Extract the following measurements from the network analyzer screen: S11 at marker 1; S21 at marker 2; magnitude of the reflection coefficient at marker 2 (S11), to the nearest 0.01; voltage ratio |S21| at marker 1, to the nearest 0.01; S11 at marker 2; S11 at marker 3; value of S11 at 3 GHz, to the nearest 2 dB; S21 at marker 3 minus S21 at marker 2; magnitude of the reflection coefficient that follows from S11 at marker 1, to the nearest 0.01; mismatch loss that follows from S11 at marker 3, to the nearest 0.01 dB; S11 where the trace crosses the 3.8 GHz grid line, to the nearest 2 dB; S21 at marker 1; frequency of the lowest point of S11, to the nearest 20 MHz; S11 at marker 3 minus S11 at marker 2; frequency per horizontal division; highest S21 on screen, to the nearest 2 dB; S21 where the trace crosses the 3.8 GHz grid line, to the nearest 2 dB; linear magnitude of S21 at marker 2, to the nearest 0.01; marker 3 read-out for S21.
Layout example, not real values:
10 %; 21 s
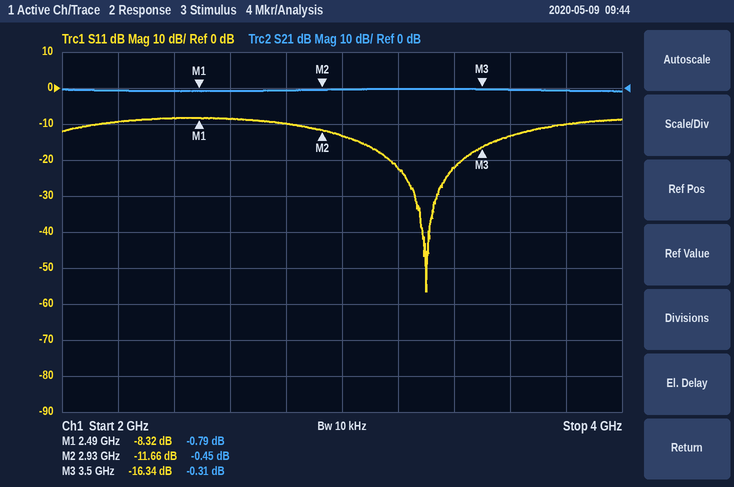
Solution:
-8.32 dB; -0.45 dB; 0.26; 0.91; -11.66 dB; -16.34 dB; -14 dB; 0.14 dB; 0.38; 0.10 dB; -10 dB; -0.79 dB; 3.30 GHz; -4.68 dB; 200 MHz; 0 dB; 0 dB; 0.95; -0.31 dB
